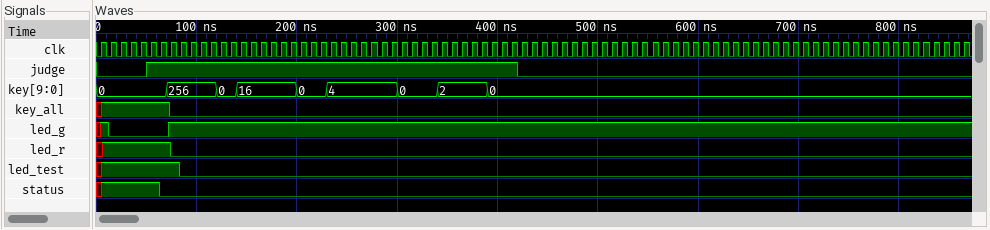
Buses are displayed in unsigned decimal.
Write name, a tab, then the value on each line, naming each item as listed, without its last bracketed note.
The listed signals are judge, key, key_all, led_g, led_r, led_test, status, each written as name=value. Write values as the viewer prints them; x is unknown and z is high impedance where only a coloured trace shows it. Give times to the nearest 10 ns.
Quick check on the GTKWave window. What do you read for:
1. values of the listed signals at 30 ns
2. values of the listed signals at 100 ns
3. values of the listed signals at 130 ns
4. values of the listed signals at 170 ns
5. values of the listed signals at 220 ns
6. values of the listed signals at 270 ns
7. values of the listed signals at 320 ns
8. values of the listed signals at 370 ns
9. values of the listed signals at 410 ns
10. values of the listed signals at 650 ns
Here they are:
values of the listed signals at 30 ns	judge=0, key=0, key_all=1, led_g=0, led_r=1, led_test=1, status=1
values of the listed signals at 100 ns	judge=1, key=256, key_all=0, led_g=1, led_r=0, led_test=0, status=0
values of the listed signals at 130 ns	judge=1, key=0, key_all=0, led_g=1, led_r=0, led_test=0, status=0
values of the listed signals at 170 ns	judge=1, key=16, key_all=0, led_g=1, led_r=0, led_test=0, status=0
values of the listed signals at 220 ns	judge=1, key=0, key_all=0, led_g=1, led_r=0, led_test=0, status=0
values of the listed signals at 270 ns	judge=1, key=4, key_all=0, led_g=1, led_r=0, led_test=0, status=0
values of the listed signals at 320 ns	judge=1, key=0, key_all=0, led_g=1, led_r=0, led_test=0, status=0
values of the listed signals at 370 ns	judge=1, key=2, key_all=0, led_g=1, led_r=0, led_test=0, status=0
values of the listed signals at 410 ns	judge=1, key=0, key_all=0, led_g=1, led_r=0, led_test=0, status=0
values of the listed signals at 650 ns	judge=0, key=0, key_all=0, led_g=1, led_r=0, led_test=0, status=0
